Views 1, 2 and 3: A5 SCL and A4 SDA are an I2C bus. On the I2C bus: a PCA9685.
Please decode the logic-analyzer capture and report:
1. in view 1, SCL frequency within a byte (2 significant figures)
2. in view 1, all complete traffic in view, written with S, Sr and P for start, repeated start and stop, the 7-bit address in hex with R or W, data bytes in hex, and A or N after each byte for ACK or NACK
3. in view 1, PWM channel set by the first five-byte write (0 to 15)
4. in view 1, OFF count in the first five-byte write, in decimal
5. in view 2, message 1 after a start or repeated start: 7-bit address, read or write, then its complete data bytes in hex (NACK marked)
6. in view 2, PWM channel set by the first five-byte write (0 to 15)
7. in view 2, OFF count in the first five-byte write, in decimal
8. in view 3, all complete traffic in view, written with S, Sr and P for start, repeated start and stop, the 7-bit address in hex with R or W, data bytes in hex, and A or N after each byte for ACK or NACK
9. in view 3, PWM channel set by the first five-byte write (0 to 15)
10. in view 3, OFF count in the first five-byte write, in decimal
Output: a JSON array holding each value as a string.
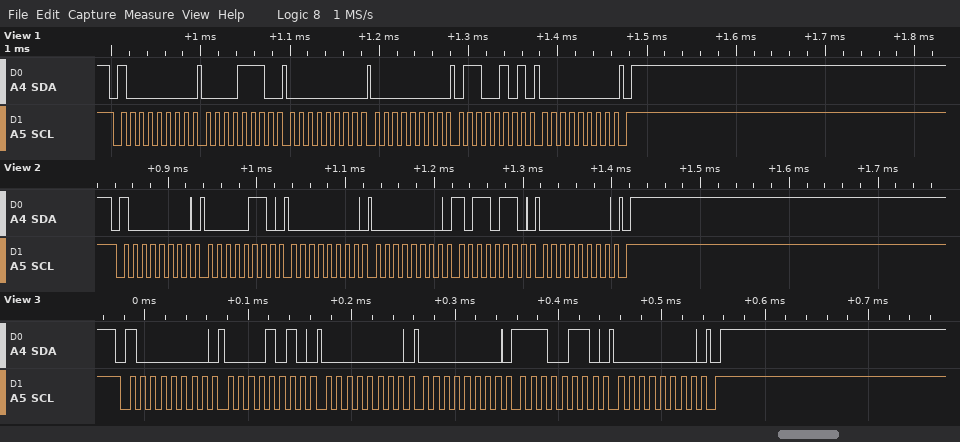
["100 kHz", "S 40W A 0E A 00 A 00 A 65 A 00 A P", "2", "101", "0x40 write: 06 00 00 B6 00", "0", "182", "S 40W A 0A A 00 A 00 A E6 A 00 A P", "1", "230"]
